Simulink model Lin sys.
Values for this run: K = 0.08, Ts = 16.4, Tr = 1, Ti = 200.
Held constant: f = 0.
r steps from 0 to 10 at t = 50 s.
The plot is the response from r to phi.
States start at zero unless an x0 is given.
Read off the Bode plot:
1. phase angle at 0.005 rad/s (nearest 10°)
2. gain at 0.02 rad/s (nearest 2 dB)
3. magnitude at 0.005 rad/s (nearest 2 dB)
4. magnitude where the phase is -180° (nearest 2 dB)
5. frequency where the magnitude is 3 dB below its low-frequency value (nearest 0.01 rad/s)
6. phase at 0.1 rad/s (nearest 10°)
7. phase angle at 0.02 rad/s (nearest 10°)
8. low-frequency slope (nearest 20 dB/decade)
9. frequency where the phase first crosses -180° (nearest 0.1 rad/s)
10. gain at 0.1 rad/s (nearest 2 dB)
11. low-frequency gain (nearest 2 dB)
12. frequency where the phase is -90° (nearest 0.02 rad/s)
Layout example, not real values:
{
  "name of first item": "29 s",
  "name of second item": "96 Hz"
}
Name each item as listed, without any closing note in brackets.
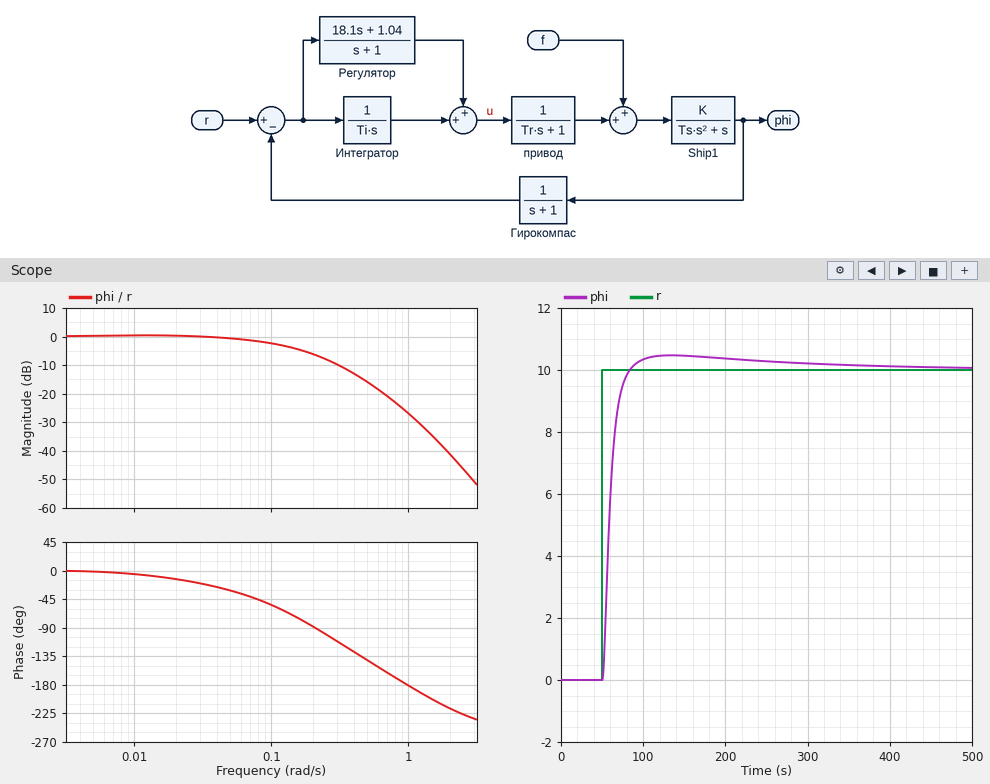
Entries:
{
  "phase angle at 0.005 rad/s": "0°",
  "gain at 0.02 rad/s": "0 dB",
  "magnitude at 0.005 rad/s": "0 dB",
  "magnitude where the phase is -180°": "-26 dB",
  "frequency where the magnitude is 3 dB below its low-frequency value": "0.11 rad/s",
  "phase at 0.1 rad/s": "-50°",
  "phase angle at 0.02 rad/s": "-10°",
  "low-frequency slope": "0 dB/decade",
  "frequency where the phase first crosses -180°": "1.0 rad/s",
  "gain at 0.1 rad/s": "-2 dB",
  "low-frequency gain": "0 dB",
  "frequency where the phase is -90°": "0.20 rad/s"
}
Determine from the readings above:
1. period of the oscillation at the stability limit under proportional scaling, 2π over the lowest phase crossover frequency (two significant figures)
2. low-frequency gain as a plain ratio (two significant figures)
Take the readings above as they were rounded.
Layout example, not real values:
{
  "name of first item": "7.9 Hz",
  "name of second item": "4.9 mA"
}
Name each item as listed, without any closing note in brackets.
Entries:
{
  "period of the oscillation at the stability limit under proportional scaling, 2π over the lowest phase crossover frequency": "6.3 s",
  "low-frequency gain as a plain ratio": "1.0"
}
